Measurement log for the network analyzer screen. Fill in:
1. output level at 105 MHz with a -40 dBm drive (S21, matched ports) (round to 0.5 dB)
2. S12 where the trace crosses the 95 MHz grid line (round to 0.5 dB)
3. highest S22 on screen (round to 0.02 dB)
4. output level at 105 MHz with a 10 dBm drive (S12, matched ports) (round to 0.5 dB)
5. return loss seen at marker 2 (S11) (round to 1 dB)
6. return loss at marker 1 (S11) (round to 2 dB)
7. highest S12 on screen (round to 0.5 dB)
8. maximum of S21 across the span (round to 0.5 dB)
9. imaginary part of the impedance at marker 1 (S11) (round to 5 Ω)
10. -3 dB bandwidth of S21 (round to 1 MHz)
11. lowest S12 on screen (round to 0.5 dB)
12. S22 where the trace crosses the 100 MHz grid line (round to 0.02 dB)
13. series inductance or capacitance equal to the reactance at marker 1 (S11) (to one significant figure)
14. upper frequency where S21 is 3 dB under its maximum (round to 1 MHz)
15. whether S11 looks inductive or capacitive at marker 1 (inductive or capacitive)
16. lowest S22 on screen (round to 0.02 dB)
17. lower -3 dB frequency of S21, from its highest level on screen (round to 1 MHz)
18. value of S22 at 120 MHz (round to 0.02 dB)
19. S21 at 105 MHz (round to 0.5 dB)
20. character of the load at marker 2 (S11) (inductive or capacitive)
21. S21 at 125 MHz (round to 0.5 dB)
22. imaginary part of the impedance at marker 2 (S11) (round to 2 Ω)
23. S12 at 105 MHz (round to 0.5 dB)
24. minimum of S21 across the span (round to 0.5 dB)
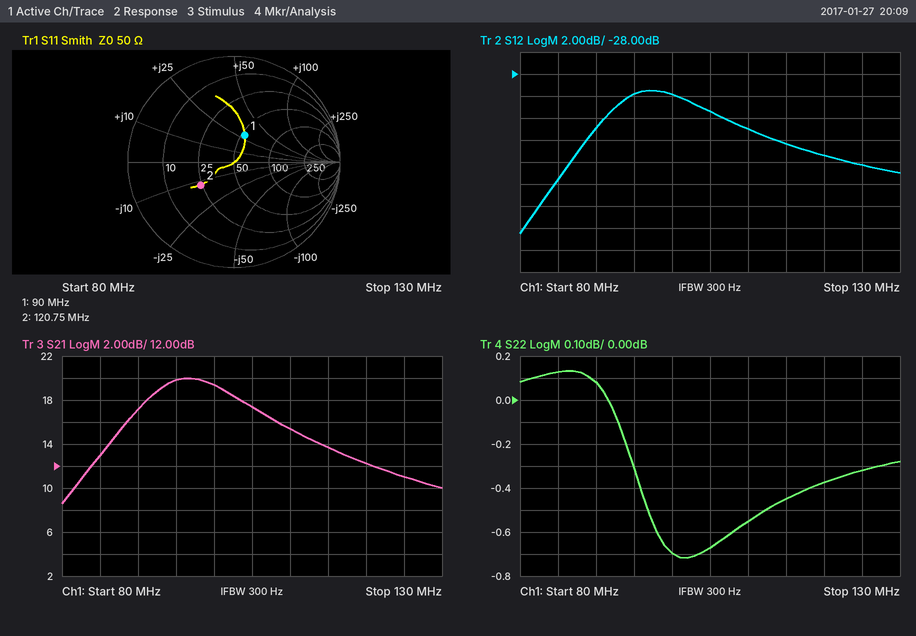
-22.5 dBm
-30.0 dB
0.14 dB
-21.5 dBm
8 dB
12 dB
-29.5 dB
20.0 dB
+30 Ω
16 MHz
-42.5 dB
-0.70 dB
50 nH
106 MHz
inductive
-0.72 dB
90 MHz
-0.38 dB
17.5 dB
capacitive
11.0 dB
-12 Ω
-31.5 dB
8.5 dB
